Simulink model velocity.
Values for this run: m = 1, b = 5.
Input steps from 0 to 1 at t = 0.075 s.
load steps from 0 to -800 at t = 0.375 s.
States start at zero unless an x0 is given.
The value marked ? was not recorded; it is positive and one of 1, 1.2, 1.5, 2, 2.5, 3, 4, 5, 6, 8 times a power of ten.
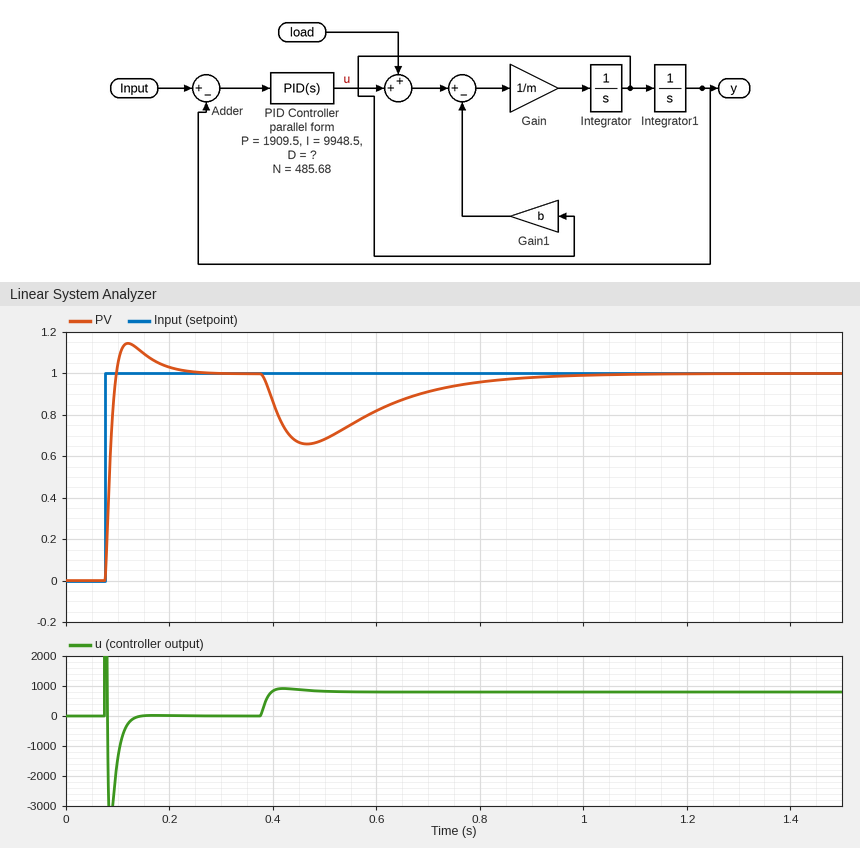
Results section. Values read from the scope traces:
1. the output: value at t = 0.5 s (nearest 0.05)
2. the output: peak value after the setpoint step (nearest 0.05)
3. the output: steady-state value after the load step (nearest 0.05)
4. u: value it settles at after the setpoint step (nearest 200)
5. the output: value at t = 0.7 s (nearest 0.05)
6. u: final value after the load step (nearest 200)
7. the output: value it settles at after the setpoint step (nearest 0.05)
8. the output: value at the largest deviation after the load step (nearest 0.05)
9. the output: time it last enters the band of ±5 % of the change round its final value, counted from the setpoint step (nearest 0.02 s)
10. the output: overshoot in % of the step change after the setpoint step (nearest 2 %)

0.70
1.15
1.00
0
0.90
800
1.00
0.65
0.10 s
14 %
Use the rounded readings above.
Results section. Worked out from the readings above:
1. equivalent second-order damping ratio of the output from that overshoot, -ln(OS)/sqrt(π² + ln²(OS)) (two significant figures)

0.53
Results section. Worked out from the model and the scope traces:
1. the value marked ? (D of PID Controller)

80
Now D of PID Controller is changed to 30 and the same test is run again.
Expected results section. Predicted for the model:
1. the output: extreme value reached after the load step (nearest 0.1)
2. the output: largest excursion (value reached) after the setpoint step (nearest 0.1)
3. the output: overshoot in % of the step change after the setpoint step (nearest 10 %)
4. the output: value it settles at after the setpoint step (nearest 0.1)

0.5
1.4
40 %
1.0
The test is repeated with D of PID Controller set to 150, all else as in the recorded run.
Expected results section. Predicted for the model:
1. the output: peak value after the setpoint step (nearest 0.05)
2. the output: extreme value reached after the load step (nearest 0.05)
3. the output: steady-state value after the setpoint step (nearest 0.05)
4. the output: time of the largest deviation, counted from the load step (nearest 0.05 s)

1.05
0.70
1.00
0.15 s
